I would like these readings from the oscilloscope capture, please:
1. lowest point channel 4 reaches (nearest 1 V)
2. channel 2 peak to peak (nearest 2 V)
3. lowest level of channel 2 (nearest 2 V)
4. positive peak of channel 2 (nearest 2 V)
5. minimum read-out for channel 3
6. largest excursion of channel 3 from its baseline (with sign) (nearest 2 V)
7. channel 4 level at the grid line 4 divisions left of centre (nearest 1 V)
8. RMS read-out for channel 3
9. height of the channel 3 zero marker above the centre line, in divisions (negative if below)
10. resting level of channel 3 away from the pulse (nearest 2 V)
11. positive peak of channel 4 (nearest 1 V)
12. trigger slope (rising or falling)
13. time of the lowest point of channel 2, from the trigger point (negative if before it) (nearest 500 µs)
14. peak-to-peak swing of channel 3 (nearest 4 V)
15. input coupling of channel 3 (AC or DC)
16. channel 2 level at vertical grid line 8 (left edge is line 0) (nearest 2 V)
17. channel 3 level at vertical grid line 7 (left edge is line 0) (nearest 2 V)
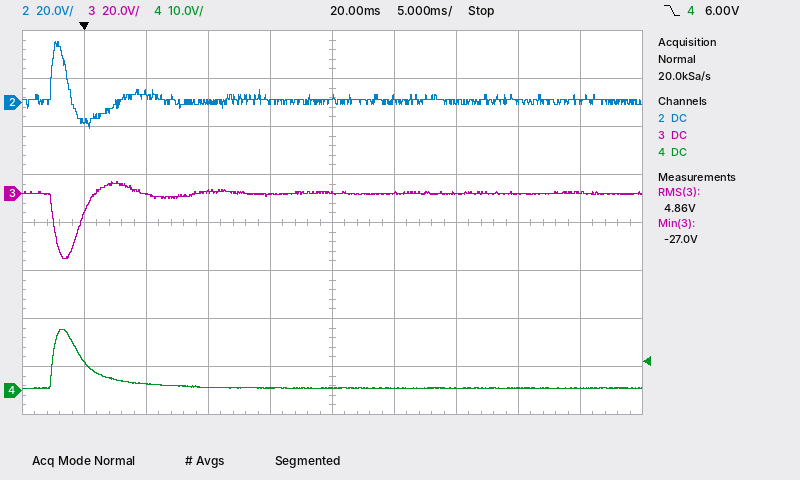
0 V
36 V
-10 V
26 V
-27.0 V
-28 V
6 V
4.86 V
+0.6 div
0 V
13 V
falling
+500 µs
32 V
DC
0 V
0 V
